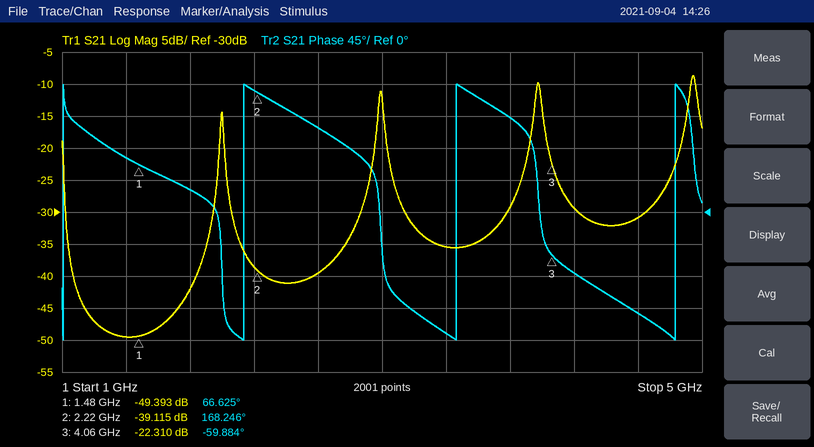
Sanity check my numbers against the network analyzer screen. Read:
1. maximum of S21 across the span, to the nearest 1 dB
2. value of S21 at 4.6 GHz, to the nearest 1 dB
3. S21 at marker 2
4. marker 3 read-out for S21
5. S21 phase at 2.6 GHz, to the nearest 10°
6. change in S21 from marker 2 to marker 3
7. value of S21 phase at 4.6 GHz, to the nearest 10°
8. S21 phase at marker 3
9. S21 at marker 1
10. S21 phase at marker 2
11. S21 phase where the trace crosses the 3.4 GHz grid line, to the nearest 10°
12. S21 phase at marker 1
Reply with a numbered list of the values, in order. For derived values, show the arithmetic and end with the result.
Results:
1. -9 dB
2. -31 dB
3. -39.115 dB
4. -22.310 dB
5. 120°
6. -22.31 − (-39.115) = 16.805 dB
7. -140°
8. -59.884°
9. -49.393 dB
10. 168.246°
11. -170°
12. 66.625°
